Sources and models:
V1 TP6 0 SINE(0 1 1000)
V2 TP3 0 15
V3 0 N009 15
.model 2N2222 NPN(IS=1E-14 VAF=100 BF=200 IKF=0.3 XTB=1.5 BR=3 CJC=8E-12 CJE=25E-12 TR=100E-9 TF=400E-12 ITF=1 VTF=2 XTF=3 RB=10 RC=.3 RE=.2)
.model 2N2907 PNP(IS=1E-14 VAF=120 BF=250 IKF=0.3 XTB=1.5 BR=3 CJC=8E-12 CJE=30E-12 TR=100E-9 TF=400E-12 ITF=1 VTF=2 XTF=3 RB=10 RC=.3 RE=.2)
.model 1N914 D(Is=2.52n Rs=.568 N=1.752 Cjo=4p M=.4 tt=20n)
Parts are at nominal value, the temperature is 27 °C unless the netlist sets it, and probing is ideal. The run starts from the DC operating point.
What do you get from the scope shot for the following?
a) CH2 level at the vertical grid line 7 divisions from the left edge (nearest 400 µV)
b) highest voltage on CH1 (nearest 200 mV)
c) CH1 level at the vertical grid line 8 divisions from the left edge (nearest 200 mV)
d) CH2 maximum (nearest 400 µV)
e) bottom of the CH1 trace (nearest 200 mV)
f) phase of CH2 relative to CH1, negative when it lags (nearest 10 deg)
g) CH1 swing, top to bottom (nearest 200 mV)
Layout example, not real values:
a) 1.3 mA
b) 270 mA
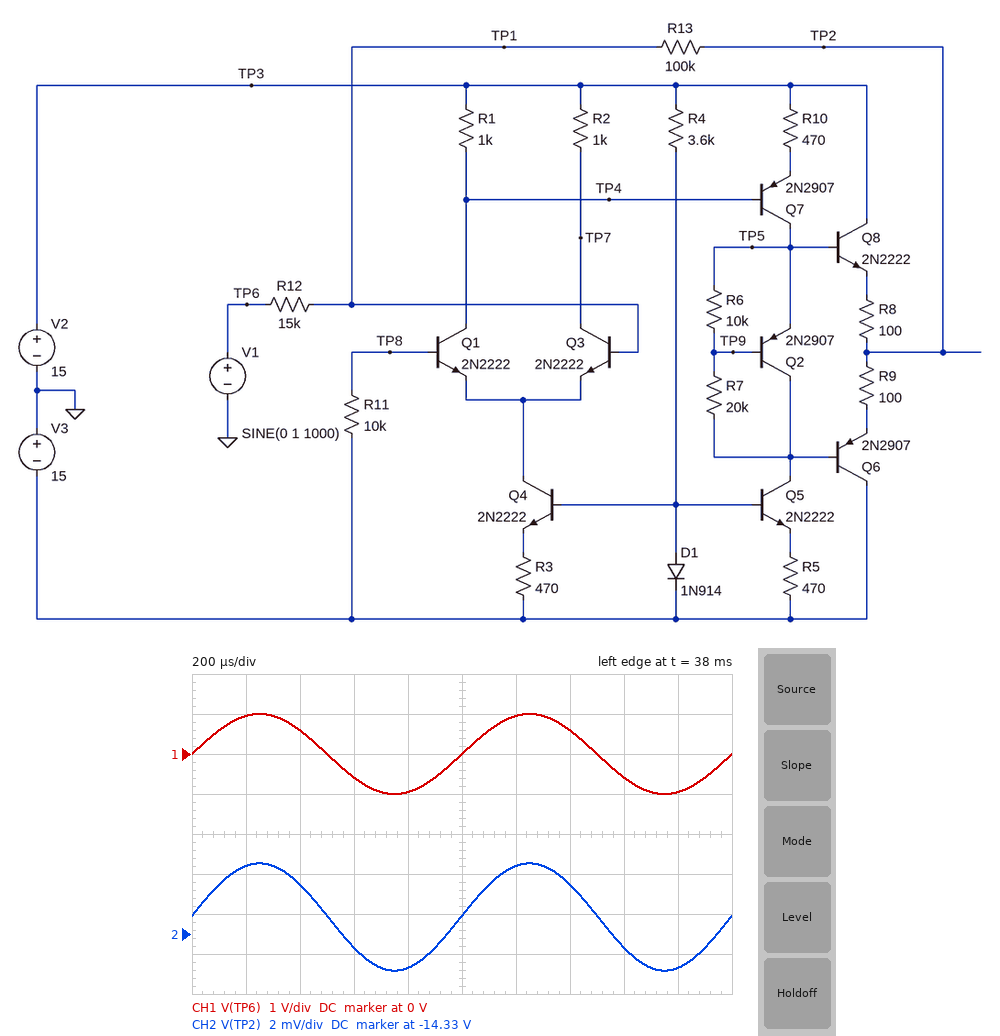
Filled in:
a) -14.3276 V
b) 1.0 V
c) -600 mV
d) -14.3264 V
e) -1.0 V
f) 0 deg
g) 2.0 V
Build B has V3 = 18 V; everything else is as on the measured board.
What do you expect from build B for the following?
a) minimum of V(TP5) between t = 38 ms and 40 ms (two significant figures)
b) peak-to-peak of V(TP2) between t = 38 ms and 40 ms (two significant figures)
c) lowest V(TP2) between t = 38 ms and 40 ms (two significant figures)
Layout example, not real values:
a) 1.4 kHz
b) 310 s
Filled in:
a) -18 V
b) 4.7 mV
c) -17 V
